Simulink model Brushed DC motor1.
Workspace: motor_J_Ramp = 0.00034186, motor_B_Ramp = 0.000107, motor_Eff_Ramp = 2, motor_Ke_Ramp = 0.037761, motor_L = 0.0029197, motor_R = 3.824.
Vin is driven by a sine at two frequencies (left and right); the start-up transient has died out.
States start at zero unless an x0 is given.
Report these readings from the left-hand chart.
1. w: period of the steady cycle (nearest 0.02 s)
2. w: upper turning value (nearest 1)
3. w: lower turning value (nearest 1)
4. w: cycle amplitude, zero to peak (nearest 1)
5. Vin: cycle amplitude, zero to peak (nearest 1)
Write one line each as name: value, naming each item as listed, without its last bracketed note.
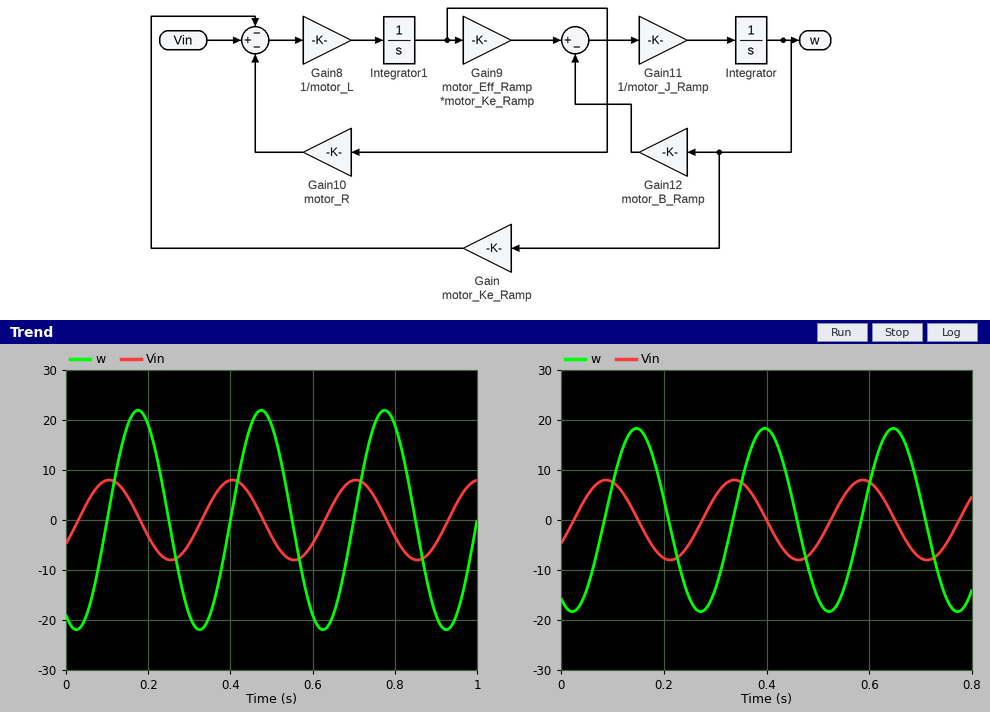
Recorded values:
w: period of the steady cycle: 0.30 s
w: upper turning value: 22
w: lower turning value: -22
w: cycle amplitude, zero to peak: 22
Vin: cycle amplitude, zero to peak: 8
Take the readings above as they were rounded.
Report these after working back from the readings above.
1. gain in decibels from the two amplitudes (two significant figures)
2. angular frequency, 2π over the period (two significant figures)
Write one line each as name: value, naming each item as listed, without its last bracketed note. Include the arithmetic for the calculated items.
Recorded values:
gain in decibels from the two amplitudes: 20 log10(22 / 8) = 8.8 dB
angular frequency, 2π over the period: 2π / 0.3 = 21 rad/s
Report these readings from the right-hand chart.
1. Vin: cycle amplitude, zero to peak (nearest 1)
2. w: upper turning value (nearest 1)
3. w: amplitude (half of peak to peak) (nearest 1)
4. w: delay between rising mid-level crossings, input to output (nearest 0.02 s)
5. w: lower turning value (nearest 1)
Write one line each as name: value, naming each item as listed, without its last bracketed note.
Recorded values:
Vin: cycle amplitude, zero to peak: 8
w: upper turning value: 18
w: amplitude (half of peak to peak): 18
w: delay between rising mid-level crossings, input to output: 0.06 s
w: lower turning value: -18
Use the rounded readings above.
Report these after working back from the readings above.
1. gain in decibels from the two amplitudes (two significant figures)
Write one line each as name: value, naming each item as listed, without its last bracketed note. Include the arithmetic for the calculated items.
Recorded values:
gain in decibels from the two amplitudes: 20 log10(18 / 8) = 7.0 dB
